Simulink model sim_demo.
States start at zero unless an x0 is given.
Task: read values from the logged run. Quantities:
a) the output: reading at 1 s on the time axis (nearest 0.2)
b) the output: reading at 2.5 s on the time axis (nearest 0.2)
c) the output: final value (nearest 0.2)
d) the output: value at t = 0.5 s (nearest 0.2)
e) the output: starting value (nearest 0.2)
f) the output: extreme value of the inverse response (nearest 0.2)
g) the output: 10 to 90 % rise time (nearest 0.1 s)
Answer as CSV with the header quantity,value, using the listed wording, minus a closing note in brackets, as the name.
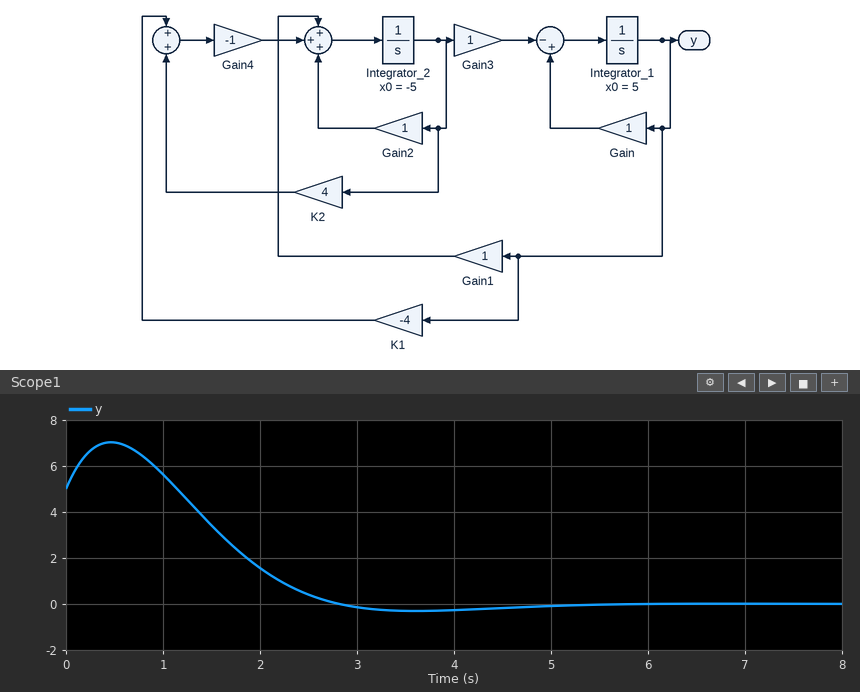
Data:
quantity,value
the output: reading at 1 s on the time axis,5.6
the output: reading at 2.5 s on the time axis,0.4
the output: final value,0.0
the output: value at t = 0.5 s,7.0
the output: starting value,5.0
the output: extreme value of the inverse response,7.0
the output: 10 to 90 % rise time,1.2 s
